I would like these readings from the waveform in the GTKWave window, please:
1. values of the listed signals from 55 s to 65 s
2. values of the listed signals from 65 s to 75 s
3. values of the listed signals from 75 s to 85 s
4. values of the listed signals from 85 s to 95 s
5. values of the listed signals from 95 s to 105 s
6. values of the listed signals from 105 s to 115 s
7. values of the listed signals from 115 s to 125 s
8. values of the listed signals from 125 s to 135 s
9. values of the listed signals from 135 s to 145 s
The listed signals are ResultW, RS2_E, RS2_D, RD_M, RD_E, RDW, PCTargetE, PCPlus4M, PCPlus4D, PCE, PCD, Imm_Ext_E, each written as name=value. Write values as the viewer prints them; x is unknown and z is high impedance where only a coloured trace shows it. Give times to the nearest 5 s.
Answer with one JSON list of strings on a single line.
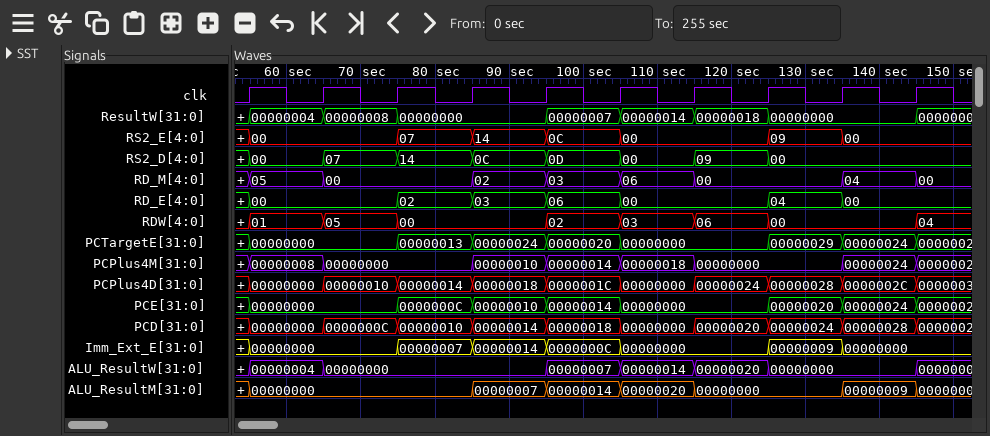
["ResultW=00000004, RS2_E=00, RS2_D=00, RD_M=05, RD_E=00, RDW=01, PCTargetE=00000000, PCPlus4M=00000008, PCPlus4D=00000000, PCE=00000000, PCD=00000000, Imm_Ext_E=00000000", "ResultW=00000008, RS2_E=00, RS2_D=07, RD_M=00, RD_E=00, RDW=05, PCTargetE=00000000, PCPlus4M=00000000, PCPlus4D=00000010, PCE=00000000, PCD=0000000C, Imm_Ext_E=00000000", "ResultW=00000000, RS2_E=07, RS2_D=14, RD_M=00, RD_E=02, RDW=00, PCTargetE=00000013, PCPlus4M=00000000, PCPlus4D=00000014, PCE=0000000C, PCD=00000010, Imm_Ext_E=00000007", "ResultW=00000000, RS2_E=14, RS2_D=0C, RD_M=02, RD_E=03, RDW=00, PCTargetE=00000024, PCPlus4M=00000010, PCPlus4D=00000018, PCE=00000010, PCD=00000014, Imm_Ext_E=00000014", "ResultW=00000007, RS2_E=0C, RS2_D=0D, RD_M=03, RD_E=06, RDW=02, PCTargetE=00000020, PCPlus4M=00000014, PCPlus4D=0000001C, PCE=00000014, PCD=00000018, Imm_Ext_E=0000000C", "ResultW=00000014, RS2_E=00, RS2_D=00, RD_M=06, RD_E=00, RDW=03, PCTargetE=00000000, PCPlus4M=00000018, PCPlus4D=00000000, PCE=00000000, PCD=00000000, Imm_Ext_E=00000000", "ResultW=00000018, RS2_E=00, RS2_D=09, RD_M=00, RD_E=00, RDW=06, PCTargetE=00000000, PCPlus4M=00000000, PCPlus4D=00000024, PCE=00000000, PCD=00000020, Imm_Ext_E=00000000", "ResultW=00000000, RS2_E=09, RS2_D=00, RD_M=00, RD_E=04, RDW=00, PCTargetE=00000029, PCPlus4M=00000000, PCPlus4D=00000028, PCE=00000020, PCD=00000024, Imm_Ext_E=00000009", "ResultW=00000000, RS2_E=00, RS2_D=00, RD_M=04, RD_E=00, RDW=00, PCTargetE=00000024, PCPlus4M=00000024, PCPlus4D=0000002C, PCE=00000024, PCD=00000028, Imm_Ext_E=00000000"]
